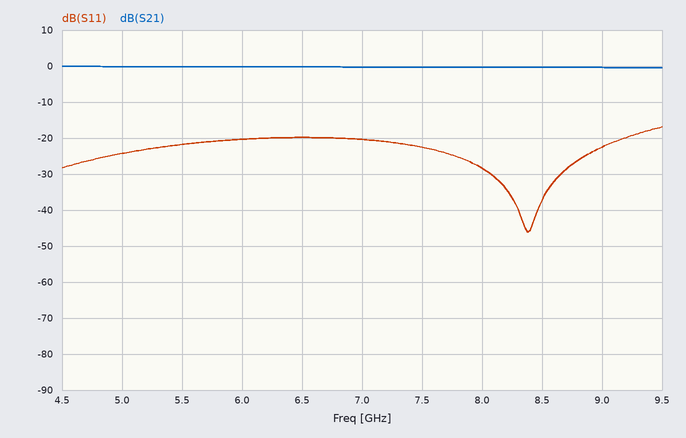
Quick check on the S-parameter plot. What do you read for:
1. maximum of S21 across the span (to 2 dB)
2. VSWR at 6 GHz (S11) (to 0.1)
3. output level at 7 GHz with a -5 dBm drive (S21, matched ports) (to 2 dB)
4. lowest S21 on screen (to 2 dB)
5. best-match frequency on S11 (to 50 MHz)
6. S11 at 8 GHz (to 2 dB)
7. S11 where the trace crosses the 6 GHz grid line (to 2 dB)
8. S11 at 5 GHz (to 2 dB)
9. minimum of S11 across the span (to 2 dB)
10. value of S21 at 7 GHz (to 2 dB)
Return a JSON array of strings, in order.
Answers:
["0 dB", "1.2", "-6 dBm", "0 dB", "8.40 GHz", "-28 dB", "-20 dB", "-24 dB", "-46 dB", "0 dB"]
